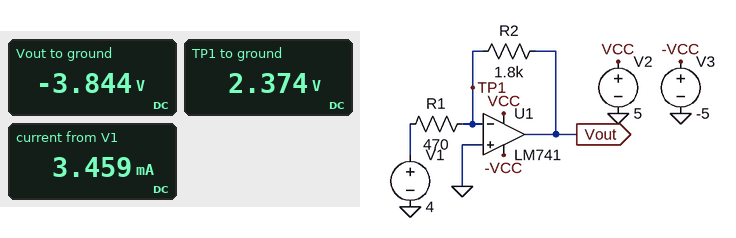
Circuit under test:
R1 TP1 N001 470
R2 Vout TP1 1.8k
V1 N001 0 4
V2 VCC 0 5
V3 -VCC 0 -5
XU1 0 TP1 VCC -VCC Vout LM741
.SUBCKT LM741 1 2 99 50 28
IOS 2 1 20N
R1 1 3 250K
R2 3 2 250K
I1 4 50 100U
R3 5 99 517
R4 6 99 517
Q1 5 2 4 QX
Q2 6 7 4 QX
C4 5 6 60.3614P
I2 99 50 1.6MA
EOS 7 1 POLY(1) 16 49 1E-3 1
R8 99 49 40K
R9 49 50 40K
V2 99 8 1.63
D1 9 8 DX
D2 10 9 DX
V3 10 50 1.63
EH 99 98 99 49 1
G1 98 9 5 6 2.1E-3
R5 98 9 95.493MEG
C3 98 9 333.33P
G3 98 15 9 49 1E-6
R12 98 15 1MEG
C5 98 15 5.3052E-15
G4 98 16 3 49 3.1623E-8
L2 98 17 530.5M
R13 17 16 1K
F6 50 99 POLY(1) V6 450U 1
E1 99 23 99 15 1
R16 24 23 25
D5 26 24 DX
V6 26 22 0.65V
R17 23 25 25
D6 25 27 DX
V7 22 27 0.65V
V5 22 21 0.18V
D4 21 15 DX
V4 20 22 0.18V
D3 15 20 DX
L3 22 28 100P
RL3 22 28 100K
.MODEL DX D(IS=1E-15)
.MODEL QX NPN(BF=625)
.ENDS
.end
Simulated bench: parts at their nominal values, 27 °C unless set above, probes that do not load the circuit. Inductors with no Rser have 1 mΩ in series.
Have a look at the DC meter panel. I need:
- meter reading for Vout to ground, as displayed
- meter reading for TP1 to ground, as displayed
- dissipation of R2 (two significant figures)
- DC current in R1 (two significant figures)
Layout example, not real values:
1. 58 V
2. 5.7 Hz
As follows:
1. -3.844 V
2. 2.374 V
3. 21 mW
4. 3.5 mA
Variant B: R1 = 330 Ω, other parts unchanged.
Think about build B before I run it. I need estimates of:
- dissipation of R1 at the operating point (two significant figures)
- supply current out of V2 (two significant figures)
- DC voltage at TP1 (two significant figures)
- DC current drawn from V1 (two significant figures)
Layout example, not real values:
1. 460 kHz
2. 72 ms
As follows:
1. 4.5 mW
2. 1.3 mA
3. 2.8 V
4. 3.7 mA
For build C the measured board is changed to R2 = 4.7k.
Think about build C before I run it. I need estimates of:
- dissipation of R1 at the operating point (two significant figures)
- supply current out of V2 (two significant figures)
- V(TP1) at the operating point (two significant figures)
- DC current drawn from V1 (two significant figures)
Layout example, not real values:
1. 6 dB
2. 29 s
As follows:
1. 1.1 mW
2. 1.3 mA
3. 3.3 V
4. 1.5 mA
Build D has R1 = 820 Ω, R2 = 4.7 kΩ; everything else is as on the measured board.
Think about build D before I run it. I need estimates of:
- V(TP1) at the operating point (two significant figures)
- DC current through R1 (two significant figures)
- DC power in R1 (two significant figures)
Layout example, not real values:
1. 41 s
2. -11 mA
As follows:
1. 2.8 V
2. 1.4 mA
3. 1.7 mW
